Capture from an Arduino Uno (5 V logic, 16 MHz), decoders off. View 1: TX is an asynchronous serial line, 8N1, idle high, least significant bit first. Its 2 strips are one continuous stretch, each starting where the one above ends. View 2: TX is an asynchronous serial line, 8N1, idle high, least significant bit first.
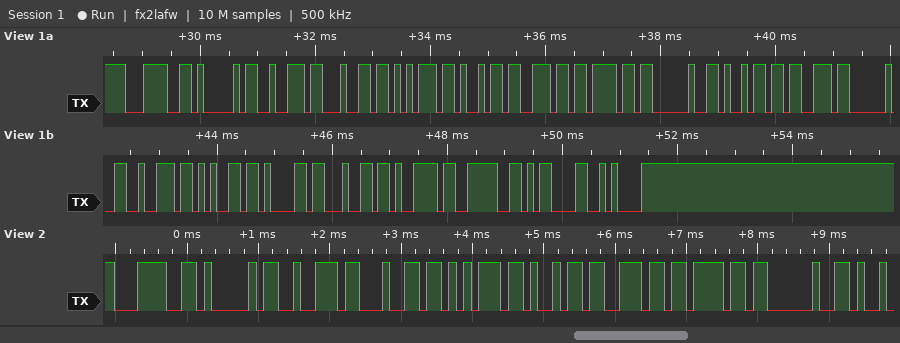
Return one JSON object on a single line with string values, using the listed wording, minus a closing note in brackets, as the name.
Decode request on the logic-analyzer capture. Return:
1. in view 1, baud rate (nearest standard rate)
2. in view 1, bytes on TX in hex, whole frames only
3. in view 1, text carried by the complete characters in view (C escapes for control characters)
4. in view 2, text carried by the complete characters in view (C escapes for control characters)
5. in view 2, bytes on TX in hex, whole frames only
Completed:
{"in view 1, baud rate": "9600 baud", "in view 1, bytes on TX in hex, whole frames only": "3C 41 72 64 75 69 6E 6F 20 69 73 20 72 65 61 64 79 3E 0D 0A", "in view 1, text carried by the complete characters in view": "\"<Arduino is ready>\\r\\n\"", "in view 2, text carried by the complete characters in view": "\"<Arduino \"", "in view 2, bytes on TX in hex, whole frames only": "3C 41 72 64 75 69 6E 6F 20"}
